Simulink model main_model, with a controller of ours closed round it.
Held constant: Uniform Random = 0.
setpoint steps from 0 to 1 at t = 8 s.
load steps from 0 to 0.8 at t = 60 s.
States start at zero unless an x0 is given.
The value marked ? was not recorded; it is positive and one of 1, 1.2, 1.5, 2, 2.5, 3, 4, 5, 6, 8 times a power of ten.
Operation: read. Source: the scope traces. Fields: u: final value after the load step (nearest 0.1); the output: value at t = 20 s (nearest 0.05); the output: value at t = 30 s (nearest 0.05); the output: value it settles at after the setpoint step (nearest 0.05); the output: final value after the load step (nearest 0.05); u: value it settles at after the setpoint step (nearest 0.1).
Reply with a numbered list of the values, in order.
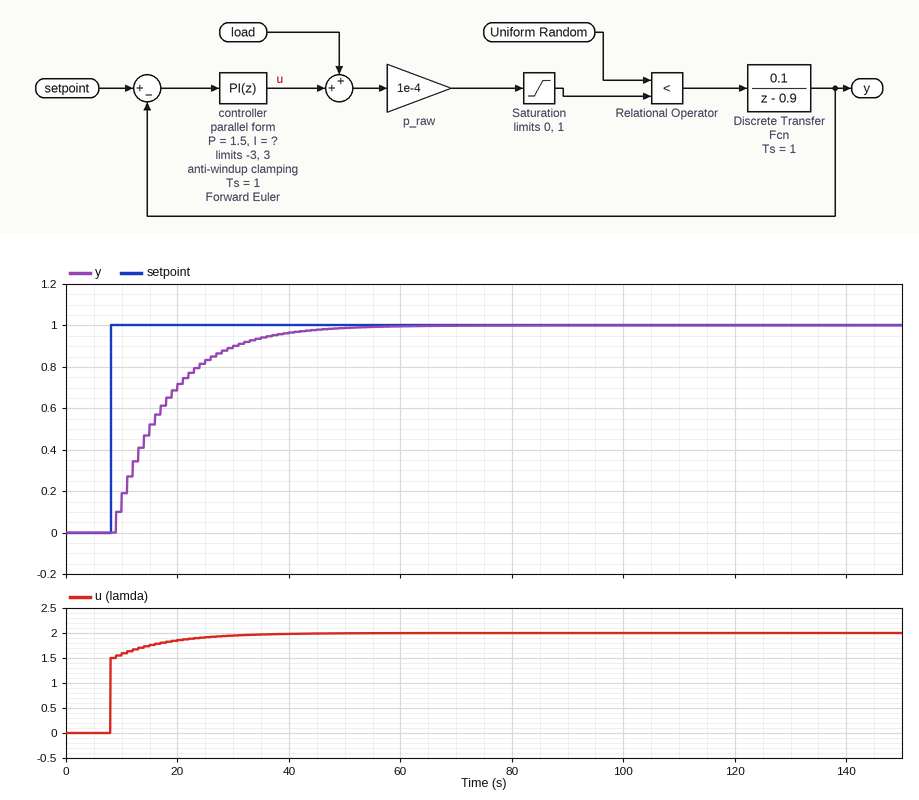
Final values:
1. 2.0
2. 0.70
3. 0.90
4. 1.00
5. 1.00
6. 2.0
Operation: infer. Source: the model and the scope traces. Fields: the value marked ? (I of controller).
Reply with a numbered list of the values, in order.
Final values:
1. 0.2
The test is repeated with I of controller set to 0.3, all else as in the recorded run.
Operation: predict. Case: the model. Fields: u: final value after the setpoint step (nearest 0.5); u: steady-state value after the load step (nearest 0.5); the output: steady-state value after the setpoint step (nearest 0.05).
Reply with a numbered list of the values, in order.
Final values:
1. 3.0
2. 3.0
3. 1.00
